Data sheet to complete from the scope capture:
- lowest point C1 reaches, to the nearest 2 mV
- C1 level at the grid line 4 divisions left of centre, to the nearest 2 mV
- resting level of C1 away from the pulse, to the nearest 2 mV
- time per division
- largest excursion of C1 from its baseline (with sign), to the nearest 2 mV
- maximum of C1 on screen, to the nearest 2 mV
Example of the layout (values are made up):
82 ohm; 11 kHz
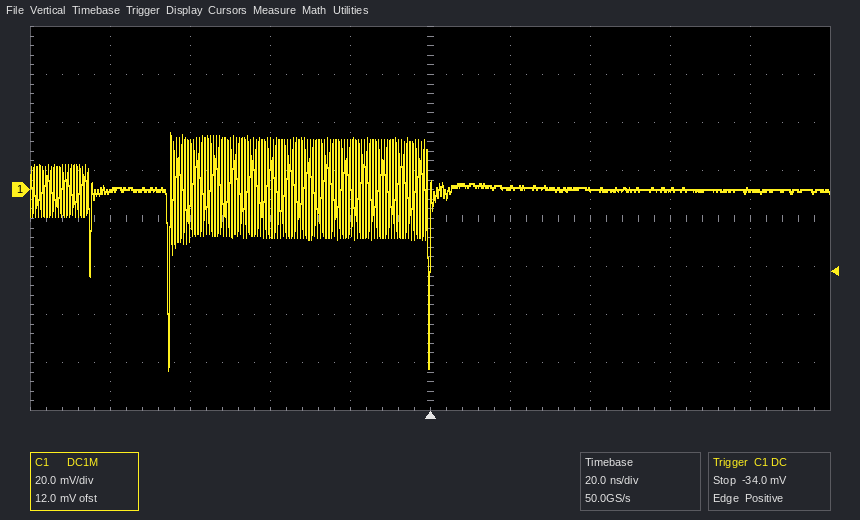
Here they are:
-76 mV; 0 mV; 0 mV; 20 ns; -76 mV; 24 mV
